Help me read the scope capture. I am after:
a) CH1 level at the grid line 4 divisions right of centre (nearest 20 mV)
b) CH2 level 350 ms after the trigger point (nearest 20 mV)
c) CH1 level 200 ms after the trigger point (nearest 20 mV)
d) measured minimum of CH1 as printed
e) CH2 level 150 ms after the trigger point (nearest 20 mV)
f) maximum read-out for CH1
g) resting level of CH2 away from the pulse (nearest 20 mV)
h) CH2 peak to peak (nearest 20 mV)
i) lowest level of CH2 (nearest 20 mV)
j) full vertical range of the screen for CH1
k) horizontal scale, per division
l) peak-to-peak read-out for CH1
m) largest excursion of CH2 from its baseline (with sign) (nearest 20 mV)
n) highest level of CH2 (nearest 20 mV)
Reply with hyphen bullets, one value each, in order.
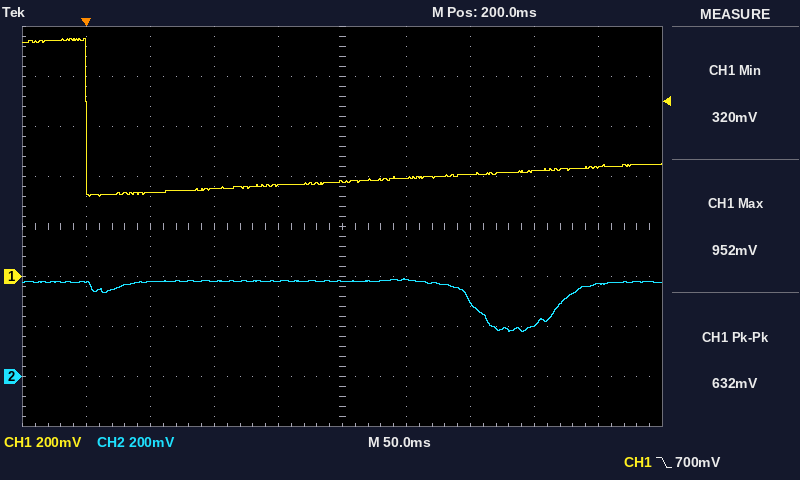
- 440 mV
- 200 mV
- 380 mV
- 320 mV
- 380 mV
- 952 mV
- 380 mV
- 220 mV
- 180 mV
- 1.6 V
- 50 ms
- 632 mV
- -200 mV
- 400 mV
